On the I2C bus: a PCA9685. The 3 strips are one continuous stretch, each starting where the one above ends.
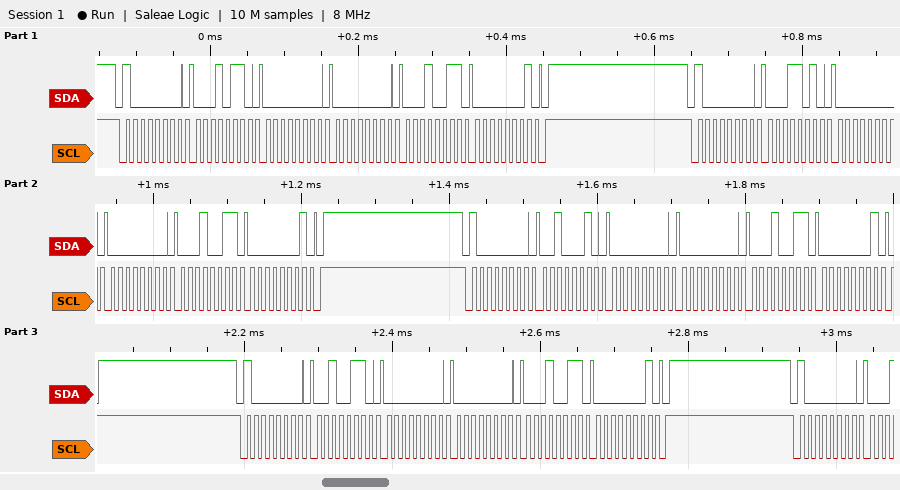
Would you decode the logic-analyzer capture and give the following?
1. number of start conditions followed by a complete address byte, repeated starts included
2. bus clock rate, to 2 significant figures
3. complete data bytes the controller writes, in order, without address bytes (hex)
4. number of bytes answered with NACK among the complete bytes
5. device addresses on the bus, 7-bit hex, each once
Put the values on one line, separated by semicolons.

5; 100 kHz; 16 00 00 13 01 1A 00 00 13 01 22 00 00 13 01 26 00 00 13 01; 0; 0x40
